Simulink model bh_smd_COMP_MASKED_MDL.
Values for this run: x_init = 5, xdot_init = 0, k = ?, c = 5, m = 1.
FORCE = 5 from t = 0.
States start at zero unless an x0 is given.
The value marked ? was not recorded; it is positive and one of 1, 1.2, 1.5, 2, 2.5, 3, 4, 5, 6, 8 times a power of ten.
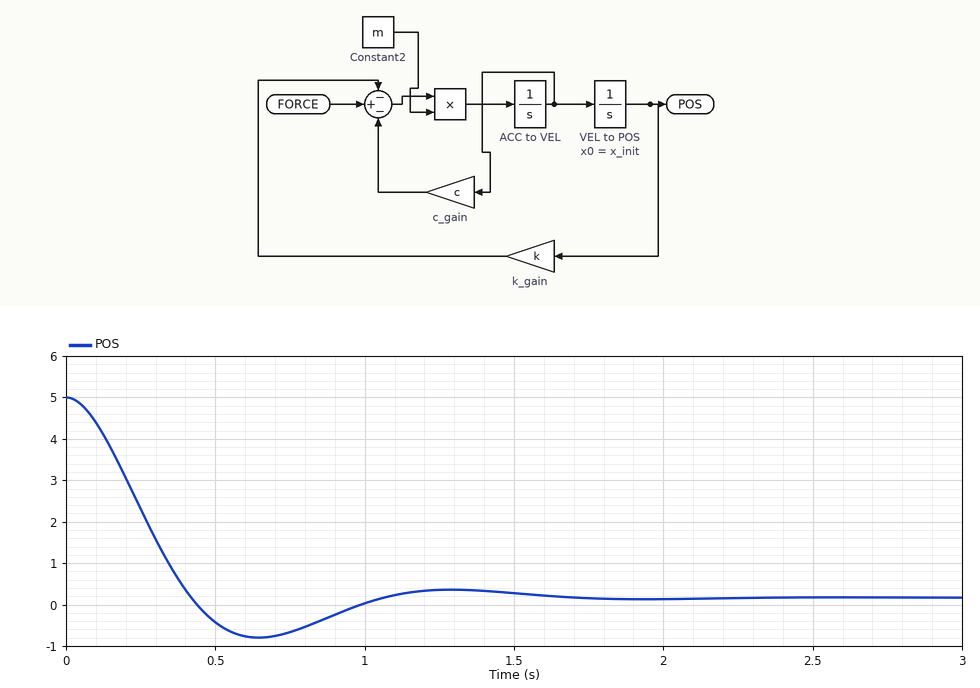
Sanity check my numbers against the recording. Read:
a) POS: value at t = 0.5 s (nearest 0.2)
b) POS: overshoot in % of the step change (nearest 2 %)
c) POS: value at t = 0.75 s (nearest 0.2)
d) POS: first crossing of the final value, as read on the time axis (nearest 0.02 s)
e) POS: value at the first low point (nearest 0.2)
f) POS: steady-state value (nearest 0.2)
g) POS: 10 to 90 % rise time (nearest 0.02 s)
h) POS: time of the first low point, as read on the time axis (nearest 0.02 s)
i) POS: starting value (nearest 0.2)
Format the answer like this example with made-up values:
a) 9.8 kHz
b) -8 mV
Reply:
a) -0.4
b) 20 %
c) -0.6
d) 0.42 s
e) -0.8
f) 0.2
g) 0.28 s
h) 0.64 s
i) 5.0
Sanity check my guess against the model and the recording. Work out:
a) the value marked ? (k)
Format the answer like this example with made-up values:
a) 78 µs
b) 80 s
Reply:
a) 30
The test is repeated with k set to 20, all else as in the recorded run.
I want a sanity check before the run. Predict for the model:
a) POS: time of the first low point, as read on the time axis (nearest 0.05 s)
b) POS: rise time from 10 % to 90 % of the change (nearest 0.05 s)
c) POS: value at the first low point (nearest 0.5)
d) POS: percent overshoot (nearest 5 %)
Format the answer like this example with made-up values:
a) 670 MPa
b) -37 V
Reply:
a) 0.85 s
b) 0.40 s
c) -0.5
d) 10 %
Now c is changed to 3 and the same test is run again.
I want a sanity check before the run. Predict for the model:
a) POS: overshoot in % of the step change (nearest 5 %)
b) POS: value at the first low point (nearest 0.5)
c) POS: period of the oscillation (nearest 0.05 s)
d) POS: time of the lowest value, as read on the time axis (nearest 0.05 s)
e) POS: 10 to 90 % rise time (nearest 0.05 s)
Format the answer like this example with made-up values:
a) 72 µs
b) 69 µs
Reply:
a) 40 %
b) -2.0
c) 1.20 s
d) 0.60 s
e) 0.25 s
